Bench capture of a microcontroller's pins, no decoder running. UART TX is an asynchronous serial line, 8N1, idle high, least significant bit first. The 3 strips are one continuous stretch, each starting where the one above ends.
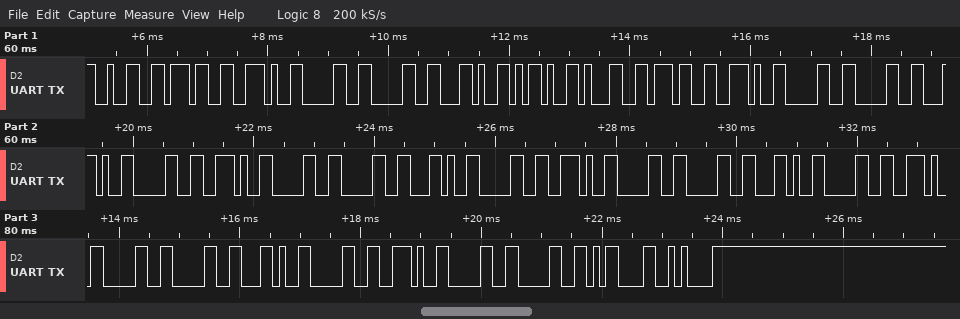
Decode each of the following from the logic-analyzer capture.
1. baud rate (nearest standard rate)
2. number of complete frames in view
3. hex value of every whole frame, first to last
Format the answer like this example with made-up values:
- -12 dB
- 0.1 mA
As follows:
- 9600 baud
- 34
- 0x32 0x37 0x2E 0x30 0x30 0x2C 0x2D 0x31 0x37 0x2E 0x30 0x30 0x2C 0x30 0x2E 0x30 0x30 0x2C 0x30 0x2E 0x30 0x30 0x2C 0x30 0x2E 0x30 0x30 0x2C 0x30 0x2E 0x30 0x30 0x0D 0x0A
